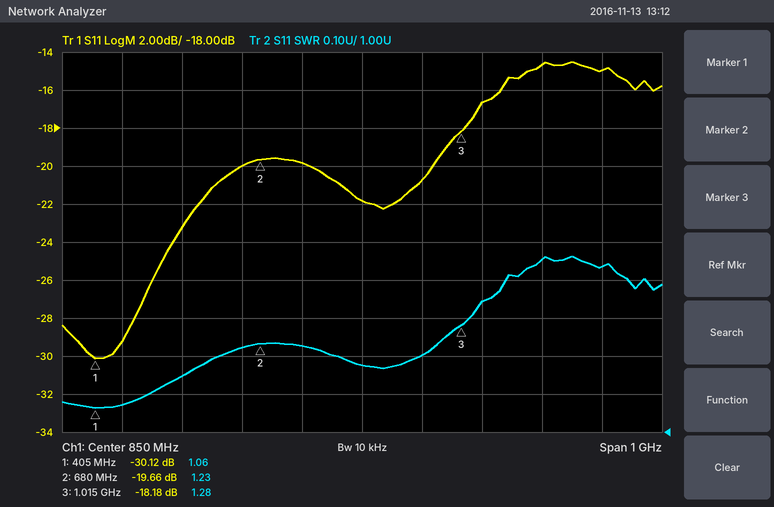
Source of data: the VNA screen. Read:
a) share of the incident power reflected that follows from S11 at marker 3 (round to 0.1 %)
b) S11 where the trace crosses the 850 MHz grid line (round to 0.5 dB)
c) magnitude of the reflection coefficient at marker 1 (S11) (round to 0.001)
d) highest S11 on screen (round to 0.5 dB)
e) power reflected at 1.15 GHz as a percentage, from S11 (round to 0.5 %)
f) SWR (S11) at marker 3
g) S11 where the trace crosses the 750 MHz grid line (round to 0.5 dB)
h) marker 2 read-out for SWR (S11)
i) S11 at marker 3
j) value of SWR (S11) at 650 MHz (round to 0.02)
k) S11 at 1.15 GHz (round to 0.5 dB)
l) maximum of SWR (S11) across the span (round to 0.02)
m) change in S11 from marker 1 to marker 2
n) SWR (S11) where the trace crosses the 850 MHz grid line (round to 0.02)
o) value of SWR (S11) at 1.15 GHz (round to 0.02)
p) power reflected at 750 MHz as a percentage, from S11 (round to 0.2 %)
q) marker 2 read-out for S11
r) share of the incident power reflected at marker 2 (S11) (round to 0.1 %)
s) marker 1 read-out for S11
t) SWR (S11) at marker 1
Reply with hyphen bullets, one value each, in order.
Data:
- 1.5 %
- -22.0 dB
- 0.031
- -14.5 dB
- 3.5 %
- 1.28
- -20.0 dB
- 1.23
- -18.18 dB
- 1.22
- -14.5 dB
- 1.46
- 10.46 dB
- 1.18
- 1.46
- 1.0 %
- -19.66 dB
- 1.1 %
- -30.12 dB
- 1.06
